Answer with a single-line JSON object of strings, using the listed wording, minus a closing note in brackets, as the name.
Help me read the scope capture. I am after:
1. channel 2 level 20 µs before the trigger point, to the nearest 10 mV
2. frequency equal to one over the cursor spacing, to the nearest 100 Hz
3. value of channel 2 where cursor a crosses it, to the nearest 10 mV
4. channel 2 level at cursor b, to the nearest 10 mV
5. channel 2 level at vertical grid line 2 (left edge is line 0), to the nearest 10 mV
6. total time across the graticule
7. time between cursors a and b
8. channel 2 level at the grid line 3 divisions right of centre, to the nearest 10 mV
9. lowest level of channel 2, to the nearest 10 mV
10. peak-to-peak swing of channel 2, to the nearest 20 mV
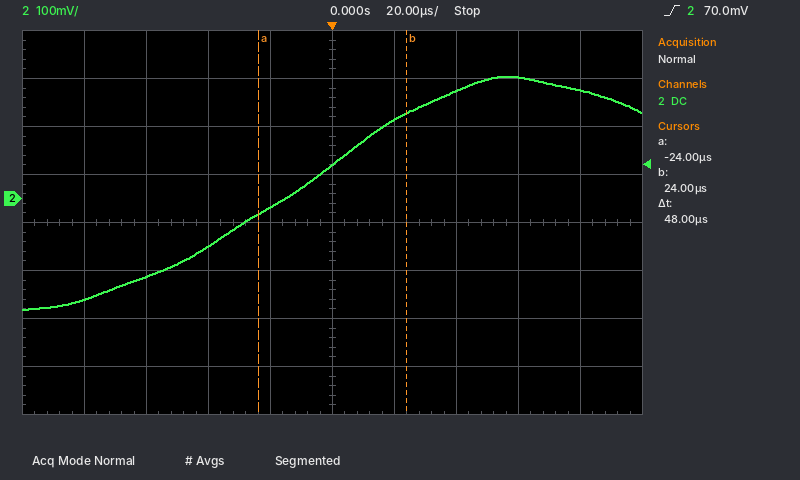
{"channel 2 level 20 µs before the trigger point, to the nearest 10 mV": "-20 mV", "frequency equal to one over the cursor spacing, to the nearest 100 Hz": "20.8 kHz", "value of channel 2 where cursor a crosses it, to the nearest 10 mV": "-30 mV", "channel 2 level at cursor b, to the nearest 10 mV": "180 mV", "channel 2 level at vertical grid line 2 (left edge is line 0), to the nearest 10 mV": "-160 mV", "total time across the graticule": "200 µs", "time between cursors a and b": "48 µs", "channel 2 level at the grid line 3 divisions right of centre, to the nearest 10 mV": "250 mV", "lowest level of channel 2, to the nearest 10 mV": "-230 mV", "peak-to-peak swing of channel 2, to the nearest 20 mV": "480 mV"}
